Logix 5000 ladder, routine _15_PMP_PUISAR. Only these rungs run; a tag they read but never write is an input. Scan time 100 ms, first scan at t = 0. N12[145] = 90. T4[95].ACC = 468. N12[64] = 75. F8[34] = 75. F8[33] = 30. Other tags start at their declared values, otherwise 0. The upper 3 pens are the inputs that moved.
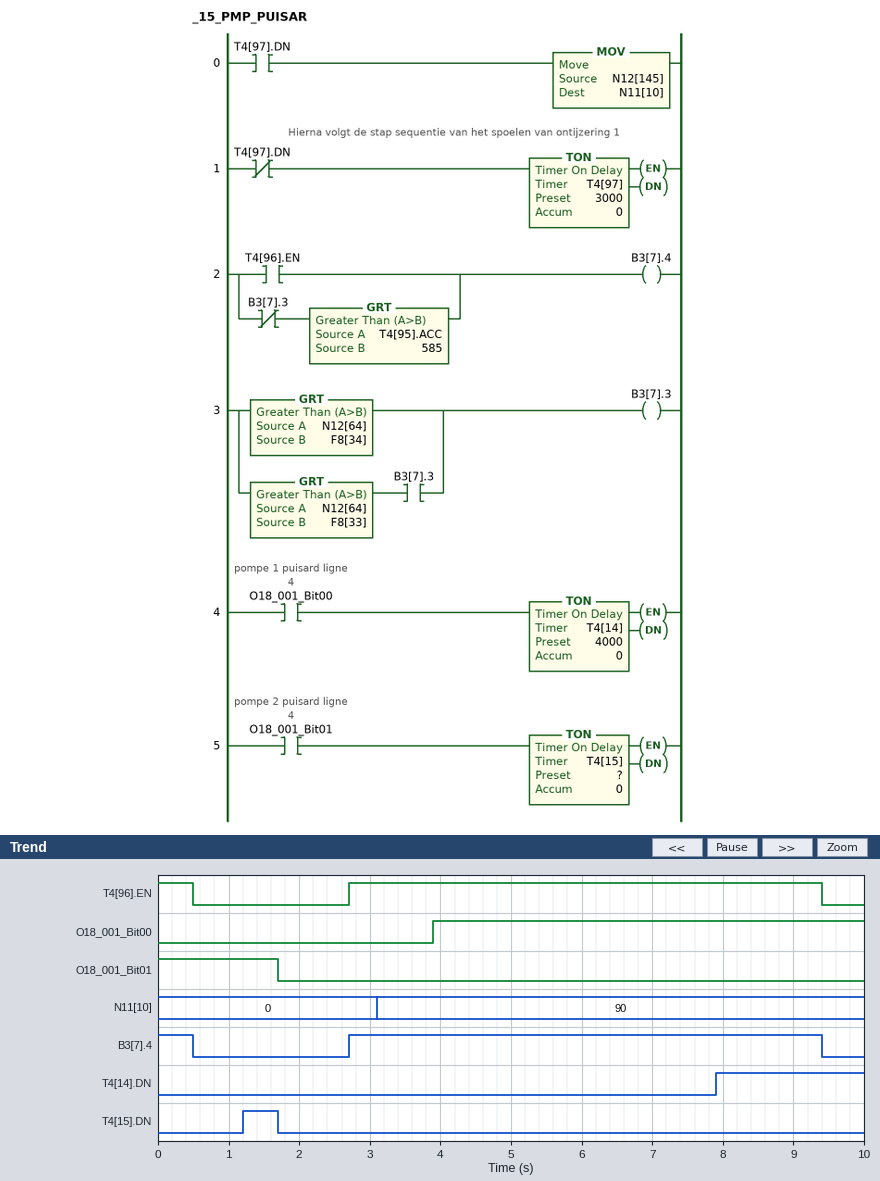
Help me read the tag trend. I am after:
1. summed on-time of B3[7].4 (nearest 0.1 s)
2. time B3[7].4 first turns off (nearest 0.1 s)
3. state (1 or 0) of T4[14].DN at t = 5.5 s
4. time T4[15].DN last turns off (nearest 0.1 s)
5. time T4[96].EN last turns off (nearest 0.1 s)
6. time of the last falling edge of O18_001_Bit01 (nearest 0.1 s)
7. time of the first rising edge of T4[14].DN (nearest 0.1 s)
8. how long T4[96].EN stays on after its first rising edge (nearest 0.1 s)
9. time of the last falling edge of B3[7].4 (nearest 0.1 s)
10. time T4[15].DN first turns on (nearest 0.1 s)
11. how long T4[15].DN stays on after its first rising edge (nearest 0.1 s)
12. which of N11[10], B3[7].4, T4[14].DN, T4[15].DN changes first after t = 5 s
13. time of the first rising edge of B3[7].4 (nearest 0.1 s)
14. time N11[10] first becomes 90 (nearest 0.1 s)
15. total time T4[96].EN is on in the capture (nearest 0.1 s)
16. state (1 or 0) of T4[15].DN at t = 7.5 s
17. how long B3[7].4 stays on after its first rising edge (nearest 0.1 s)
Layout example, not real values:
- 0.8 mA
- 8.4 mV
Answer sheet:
- 7.2 s
- 0.5 s
- 0
- 1.7 s
- 9.4 s
- 1.7 s
- 7.9 s
- 6.7 s
- 9.4 s
- 1.2 s
- 0.5 s
- T4[14].DN
- 2.7 s
- 3.1 s
- 7.2 s
- 0
- 6.7 s
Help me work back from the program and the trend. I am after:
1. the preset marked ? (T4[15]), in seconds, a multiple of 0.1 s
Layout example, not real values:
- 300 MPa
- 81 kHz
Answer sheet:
- 1.2 s
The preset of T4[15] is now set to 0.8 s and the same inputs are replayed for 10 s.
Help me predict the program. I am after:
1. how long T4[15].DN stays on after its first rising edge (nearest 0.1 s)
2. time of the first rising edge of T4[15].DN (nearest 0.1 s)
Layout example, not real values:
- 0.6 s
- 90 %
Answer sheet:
- 0.9 s
- 0.8 s
